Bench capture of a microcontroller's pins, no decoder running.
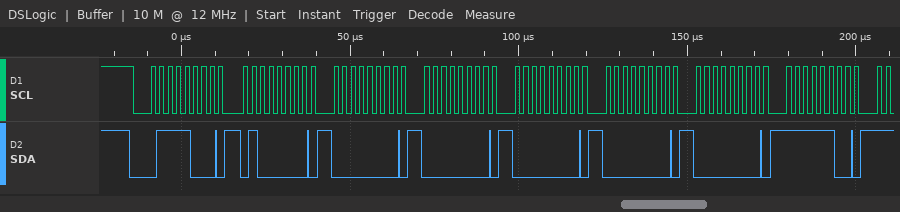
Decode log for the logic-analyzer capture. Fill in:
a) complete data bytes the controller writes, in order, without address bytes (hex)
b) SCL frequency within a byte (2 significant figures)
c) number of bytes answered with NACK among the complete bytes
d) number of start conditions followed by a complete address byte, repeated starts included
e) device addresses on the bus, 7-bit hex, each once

40 00 00 00 00 00 FC
400 kHz
0
1
0x3C
